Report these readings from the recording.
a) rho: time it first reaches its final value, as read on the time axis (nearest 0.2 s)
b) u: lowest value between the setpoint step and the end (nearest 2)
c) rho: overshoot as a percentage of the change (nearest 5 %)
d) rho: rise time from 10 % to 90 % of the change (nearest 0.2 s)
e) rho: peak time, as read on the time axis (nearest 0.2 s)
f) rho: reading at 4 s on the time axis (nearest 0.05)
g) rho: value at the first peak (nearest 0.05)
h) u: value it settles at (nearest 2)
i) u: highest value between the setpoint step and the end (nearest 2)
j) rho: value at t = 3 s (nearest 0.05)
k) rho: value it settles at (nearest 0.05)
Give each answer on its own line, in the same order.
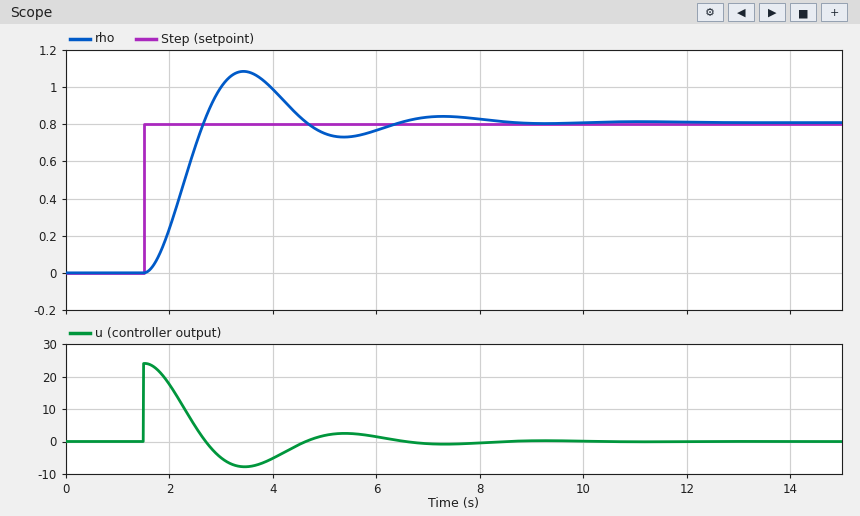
2.6 s
-8
35 %
0.8 s
3.4 s
1.00
1.10
0
24
1.00
0.80
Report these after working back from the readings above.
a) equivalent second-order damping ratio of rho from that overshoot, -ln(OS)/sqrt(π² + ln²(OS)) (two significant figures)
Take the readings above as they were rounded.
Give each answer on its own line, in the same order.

0.32
